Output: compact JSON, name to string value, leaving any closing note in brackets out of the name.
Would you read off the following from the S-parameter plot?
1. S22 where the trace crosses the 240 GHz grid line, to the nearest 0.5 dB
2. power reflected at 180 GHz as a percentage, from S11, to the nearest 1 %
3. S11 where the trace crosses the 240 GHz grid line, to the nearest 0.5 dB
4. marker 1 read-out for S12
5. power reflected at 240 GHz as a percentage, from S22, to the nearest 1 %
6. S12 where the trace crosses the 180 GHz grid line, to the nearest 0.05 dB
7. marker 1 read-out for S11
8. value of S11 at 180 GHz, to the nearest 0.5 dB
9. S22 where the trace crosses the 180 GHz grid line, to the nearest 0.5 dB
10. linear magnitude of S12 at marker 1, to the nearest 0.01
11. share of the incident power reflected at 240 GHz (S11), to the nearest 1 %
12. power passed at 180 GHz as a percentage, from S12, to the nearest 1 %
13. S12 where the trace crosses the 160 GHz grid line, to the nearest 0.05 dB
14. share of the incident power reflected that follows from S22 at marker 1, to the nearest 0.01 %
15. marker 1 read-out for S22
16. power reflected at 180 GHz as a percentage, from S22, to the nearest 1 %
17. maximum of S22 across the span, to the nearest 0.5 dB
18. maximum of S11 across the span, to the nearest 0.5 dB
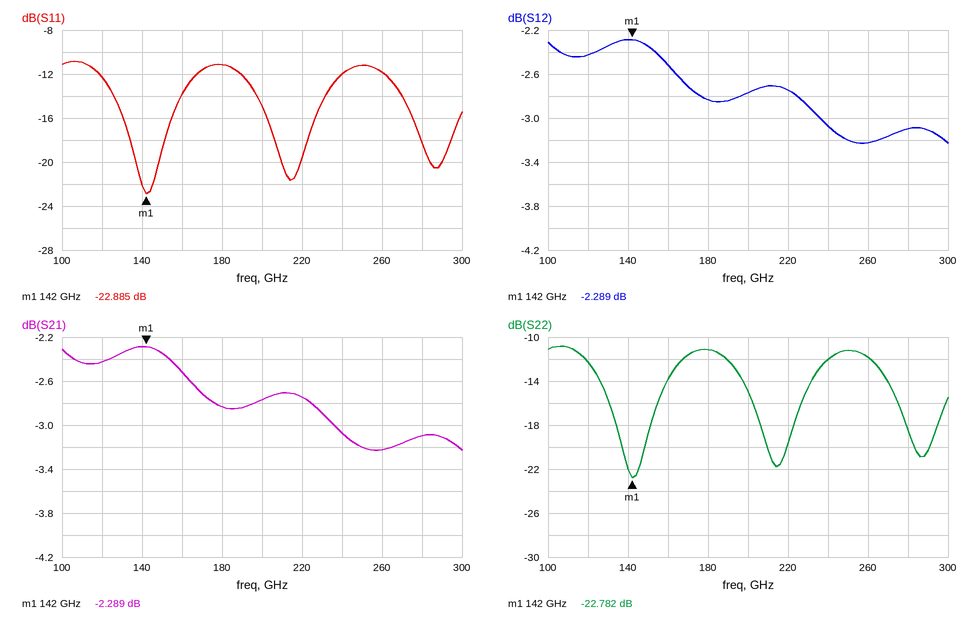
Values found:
{"S22 where the trace crosses the 240 GHz grid line, to the nearest 0.5 dB": "-12.0 dB", "power reflected at 180 GHz as a percentage, from S11, to the nearest 1 %": "8 %", "S11 where the trace crosses the 240 GHz grid line, to the nearest 0.5 dB": "-12.0 dB", "marker 1 read-out for S12": "-2.289 dB", "power reflected at 240 GHz as a percentage, from S22, to the nearest 1 %": "6 %", "S12 where the trace crosses the 180 GHz grid line, to the nearest 0.05 dB": "-2.85 dB", "marker 1 read-out for S11": "-22.885 dB", "value of S11 at 180 GHz, to the nearest 0.5 dB": "-11.0 dB", "S22 where the trace crosses the 180 GHz grid line, to the nearest 0.5 dB": "-11.0 dB", "linear magnitude of S12 at marker 1, to the nearest 0.01": "0.77", "share of the incident power reflected at 240 GHz (S11), to the nearest 1 %": "6 %", "power passed at 180 GHz as a percentage, from S12, to the nearest 1 %": "52 %", "S12 where the trace crosses the 160 GHz grid line, to the nearest 0.05 dB": "-2.50 dB", "share of the incident power reflected that follows from S22 at marker 1, to the nearest 0.01 %": "0.53 %", "marker 1 read-out for S22": "-22.782 dB", "power reflected at 180 GHz as a percentage, from S22, to the nearest 1 %": "8 %", "maximum of S22 across the span, to the nearest 0.5 dB": "-11.0 dB", "maximum of S11 across the span, to the nearest 0.5 dB": "-11.0 dB"}
